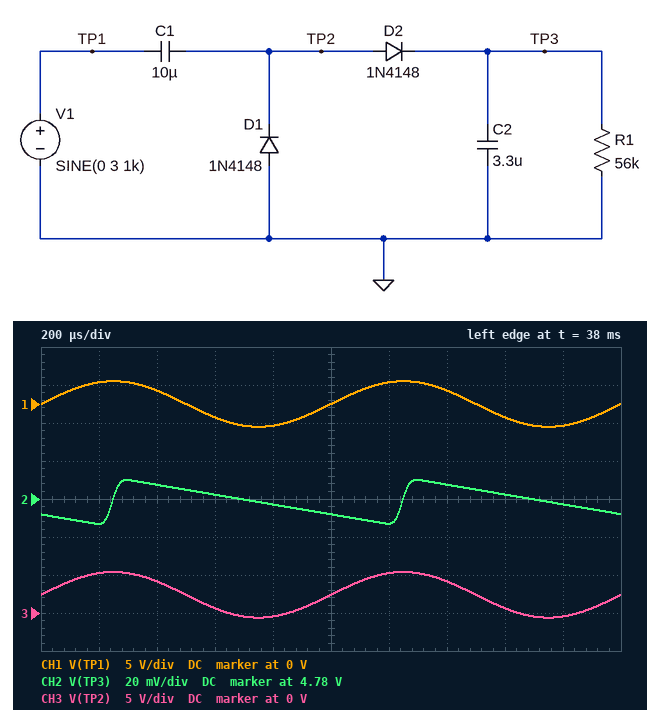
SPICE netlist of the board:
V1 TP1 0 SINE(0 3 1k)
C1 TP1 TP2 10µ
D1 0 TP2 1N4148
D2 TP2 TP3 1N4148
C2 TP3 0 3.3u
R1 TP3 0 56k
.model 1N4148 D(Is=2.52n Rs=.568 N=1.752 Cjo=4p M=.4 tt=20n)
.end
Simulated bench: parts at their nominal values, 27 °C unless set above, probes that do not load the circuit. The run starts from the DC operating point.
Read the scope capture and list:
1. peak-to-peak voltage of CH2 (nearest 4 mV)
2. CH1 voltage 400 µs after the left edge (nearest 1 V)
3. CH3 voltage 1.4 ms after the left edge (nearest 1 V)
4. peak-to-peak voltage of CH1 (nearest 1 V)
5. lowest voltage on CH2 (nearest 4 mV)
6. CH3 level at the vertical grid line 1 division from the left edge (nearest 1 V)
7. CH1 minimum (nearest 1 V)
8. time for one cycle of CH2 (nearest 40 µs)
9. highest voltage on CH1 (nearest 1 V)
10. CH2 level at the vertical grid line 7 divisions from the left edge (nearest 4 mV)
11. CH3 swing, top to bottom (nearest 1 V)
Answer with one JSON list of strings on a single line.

["24 mV", "2 V", "4 V", "6 V", "4.768 V", "5 V", "-3 V", "1.00 ms", "3 V", "4.788 V", "6 V"]
